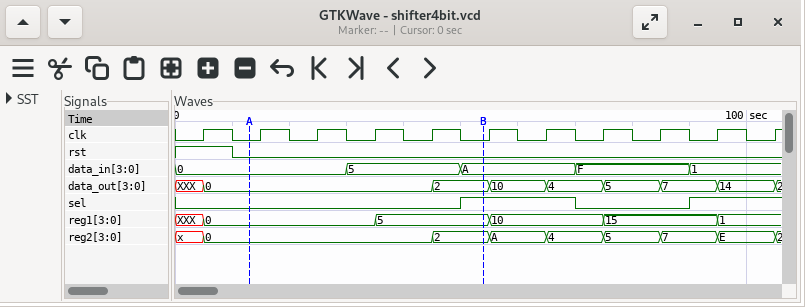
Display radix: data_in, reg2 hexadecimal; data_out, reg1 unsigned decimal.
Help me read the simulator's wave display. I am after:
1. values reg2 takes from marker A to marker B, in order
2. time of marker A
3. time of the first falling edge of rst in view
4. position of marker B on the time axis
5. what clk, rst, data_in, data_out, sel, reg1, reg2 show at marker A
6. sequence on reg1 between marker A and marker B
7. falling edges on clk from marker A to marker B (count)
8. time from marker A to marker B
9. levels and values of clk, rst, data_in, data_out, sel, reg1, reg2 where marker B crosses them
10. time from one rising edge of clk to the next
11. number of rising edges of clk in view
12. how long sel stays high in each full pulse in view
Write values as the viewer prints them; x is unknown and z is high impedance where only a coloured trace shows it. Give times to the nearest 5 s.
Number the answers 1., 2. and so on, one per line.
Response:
1. 0, 2
2. 15 s
3. 10 s
4. 55 s
5. clk=0, rst=0, data_in=0, data_out=0, sel=0, reg1=0, reg2=0
6. 0, 5
7. 4
8. 40 s
9. clk=0, rst=0, data_in=A, data_out=2, sel=1, reg1=5, reg2=2
10. 10 s
11. 11
12. 20 s
